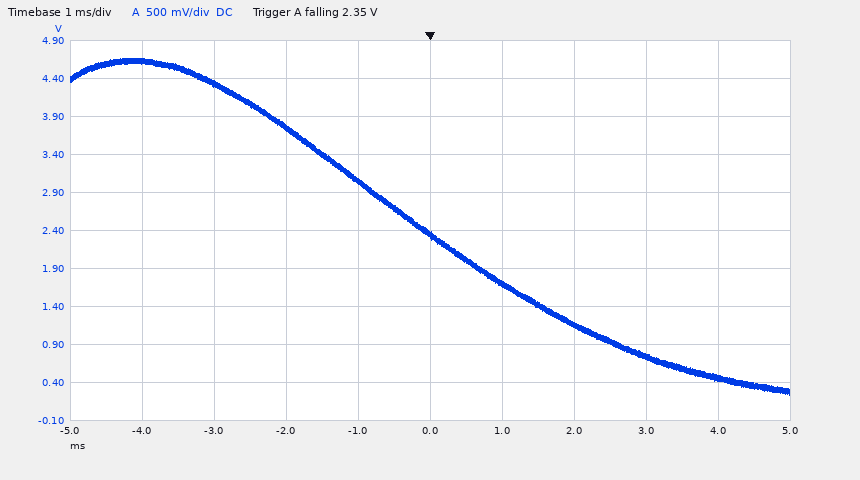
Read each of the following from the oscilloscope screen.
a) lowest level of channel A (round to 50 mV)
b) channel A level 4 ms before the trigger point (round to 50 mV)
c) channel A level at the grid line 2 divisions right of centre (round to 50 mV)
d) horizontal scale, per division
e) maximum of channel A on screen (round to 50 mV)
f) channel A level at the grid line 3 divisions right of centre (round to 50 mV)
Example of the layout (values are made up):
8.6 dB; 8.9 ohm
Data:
250 mV; 4.65 V; 1.15 V; 1 ms; 4.65 V; 750 mV
